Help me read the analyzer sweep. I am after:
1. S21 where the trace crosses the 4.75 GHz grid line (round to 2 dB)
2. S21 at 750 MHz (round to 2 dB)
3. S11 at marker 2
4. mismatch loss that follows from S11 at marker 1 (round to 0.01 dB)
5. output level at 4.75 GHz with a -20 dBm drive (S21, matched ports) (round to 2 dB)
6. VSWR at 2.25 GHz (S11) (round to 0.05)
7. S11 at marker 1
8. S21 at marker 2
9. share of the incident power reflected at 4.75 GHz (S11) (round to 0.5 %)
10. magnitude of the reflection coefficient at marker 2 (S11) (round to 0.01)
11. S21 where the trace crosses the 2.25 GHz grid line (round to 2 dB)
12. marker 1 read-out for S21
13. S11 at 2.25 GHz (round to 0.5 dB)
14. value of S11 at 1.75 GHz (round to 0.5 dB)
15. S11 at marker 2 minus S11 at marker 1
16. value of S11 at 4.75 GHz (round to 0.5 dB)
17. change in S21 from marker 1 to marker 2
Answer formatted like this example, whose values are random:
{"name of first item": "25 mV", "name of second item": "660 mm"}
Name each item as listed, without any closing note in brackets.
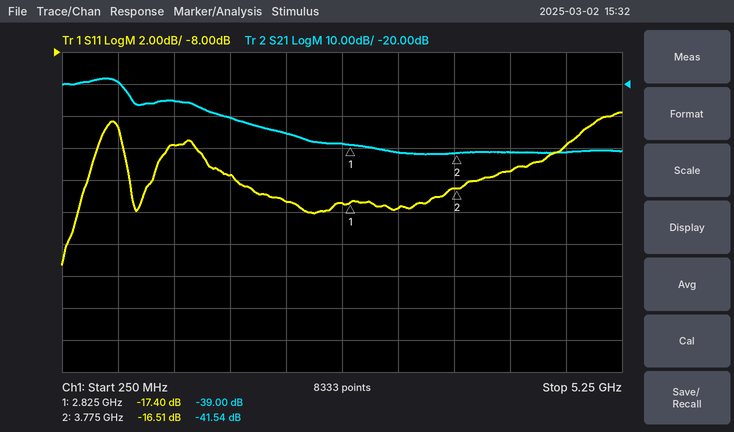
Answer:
{"S21 where the trace crosses the 4.75 GHz grid line": "-42 dB", "S21 at 750 MHz": "-20 dB", "S11 at marker 2": "-16.51 dB", "mismatch loss that follows from S11 at marker 1": "0.08 dB", "output level at 4.75 GHz with a -20 dBm drive (S21, matched ports)": "-62 dBm", "VSWR at 2.25 GHz (S11)": "1.30", "S11 at marker 1": "-17.40 dB", "S21 at marker 2": "-41.54 dB", "share of the incident power reflected at 4.75 GHz (S11)": "4.0 %", "magnitude of the reflection coefficient at marker 2 (S11)": "0.15", "S21 where the trace crosses the 2.25 GHz grid line": "-36 dB", "marker 1 read-out for S21": "-39.00 dB", "S11 at 2.25 GHz": "-17.5 dB", "value of S11 at 1.75 GHz": "-15.5 dB", "S11 at marker 2 minus S11 at marker 1": "0.89 dB", "value of S11 at 4.75 GHz": "-14.0 dB", "change in S21 from marker 1 to marker 2": "-2.54 dB"}
